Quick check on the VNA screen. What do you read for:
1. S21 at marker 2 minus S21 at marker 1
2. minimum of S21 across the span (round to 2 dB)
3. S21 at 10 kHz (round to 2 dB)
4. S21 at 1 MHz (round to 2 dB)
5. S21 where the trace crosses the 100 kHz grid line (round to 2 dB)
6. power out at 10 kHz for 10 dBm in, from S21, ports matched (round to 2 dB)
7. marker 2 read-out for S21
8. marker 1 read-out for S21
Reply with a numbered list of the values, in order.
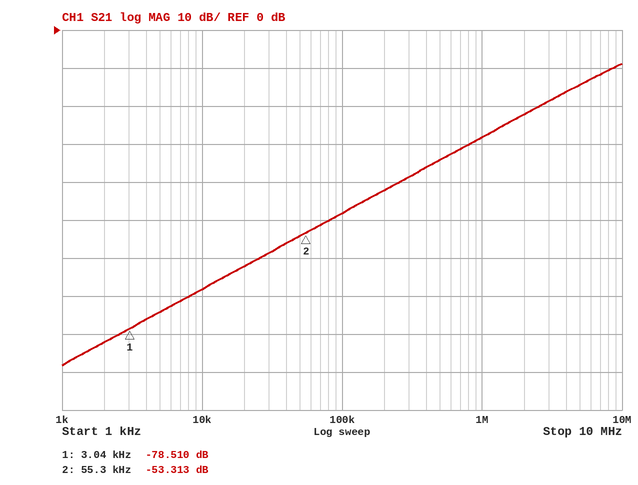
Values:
1. 25.197 dB
2. -88 dB
3. -68 dB
4. -28 dB
5. -48 dB
6. -58 dBm
7. -53.313 dB
8. -78.510 dB
